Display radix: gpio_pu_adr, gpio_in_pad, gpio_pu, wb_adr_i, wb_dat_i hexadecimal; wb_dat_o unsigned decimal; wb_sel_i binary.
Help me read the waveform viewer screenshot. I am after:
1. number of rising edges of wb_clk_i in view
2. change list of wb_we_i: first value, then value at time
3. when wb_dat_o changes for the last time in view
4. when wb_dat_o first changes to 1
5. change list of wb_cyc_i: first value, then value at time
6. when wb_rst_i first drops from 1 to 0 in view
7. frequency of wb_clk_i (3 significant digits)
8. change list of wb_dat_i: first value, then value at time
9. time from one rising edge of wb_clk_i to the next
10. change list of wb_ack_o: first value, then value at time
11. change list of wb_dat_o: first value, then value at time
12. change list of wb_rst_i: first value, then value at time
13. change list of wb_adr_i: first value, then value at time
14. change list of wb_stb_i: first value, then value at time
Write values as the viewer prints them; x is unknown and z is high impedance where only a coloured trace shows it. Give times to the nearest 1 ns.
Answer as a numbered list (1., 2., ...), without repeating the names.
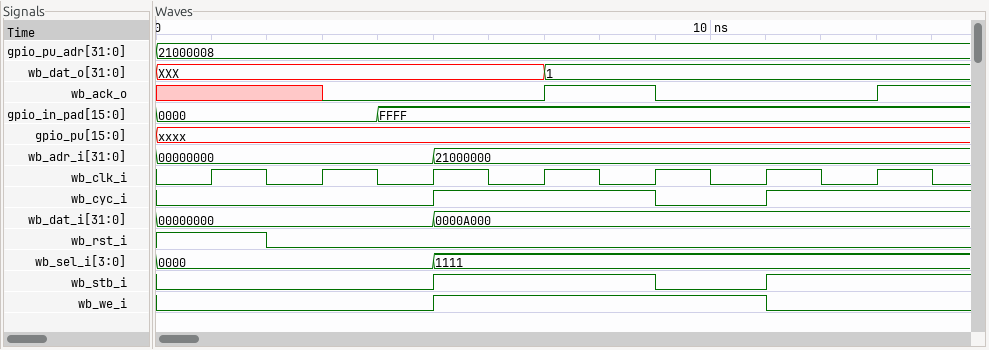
1. 7
2. 0, 1 at 5 ns, 0 at 11 ns
3. 7 ns
4. 7 ns
5. 0, 1 at 5 ns, 0 at 9 ns, 1 at 11 ns
6. 2 ns
7. 500 MHz
8. 00000000, 0000A000 at 5 ns
9. 2 ns
10. x, 0 at 3 ns, 1 at 7 ns, 0 at 9 ns, 1 at 13 ns
11. XXX, 1 at 7 ns
12. 1, 0 at 2 ns
13. 00000000, 21000000 at 5 ns
14. 0, 1 at 5 ns, 0 at 9 ns, 1 at 11 ns
